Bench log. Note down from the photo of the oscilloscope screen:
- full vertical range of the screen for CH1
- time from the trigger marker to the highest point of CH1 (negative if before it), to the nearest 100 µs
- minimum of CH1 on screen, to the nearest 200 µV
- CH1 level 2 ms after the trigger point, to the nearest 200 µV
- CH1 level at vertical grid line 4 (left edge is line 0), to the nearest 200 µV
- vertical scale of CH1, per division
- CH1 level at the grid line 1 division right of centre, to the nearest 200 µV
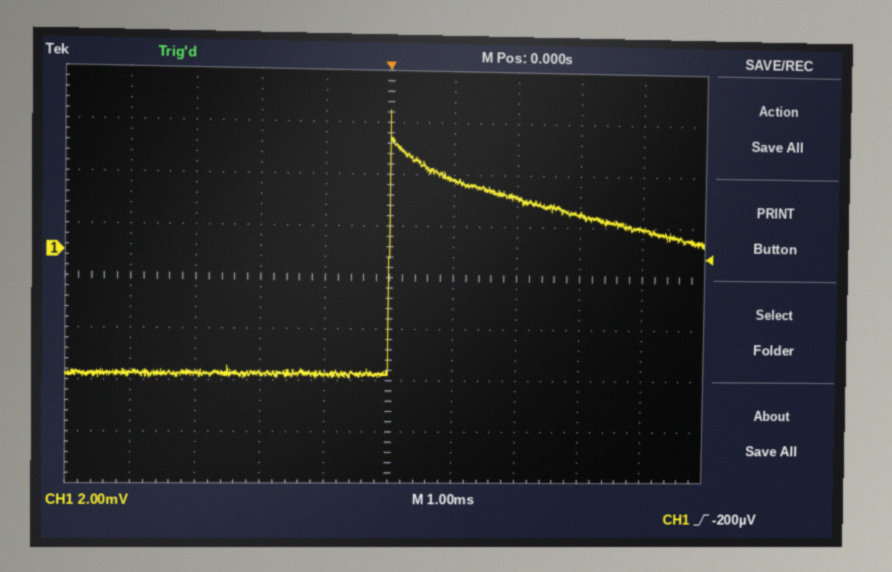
16 mV
0.0 ms
-4.8 mV
2.2 mV
-4.8 mV
2 mV
2.8 mV
